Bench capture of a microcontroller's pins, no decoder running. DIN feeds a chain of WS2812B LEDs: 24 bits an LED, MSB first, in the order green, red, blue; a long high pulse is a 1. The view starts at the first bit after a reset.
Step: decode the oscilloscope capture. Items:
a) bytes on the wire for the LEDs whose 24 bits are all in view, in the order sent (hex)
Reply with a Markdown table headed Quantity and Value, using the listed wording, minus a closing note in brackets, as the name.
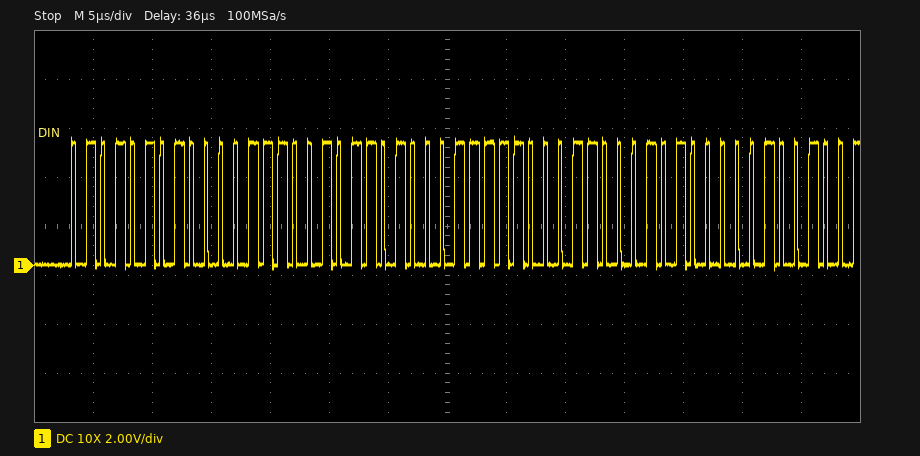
| Quantity | Value |
|---|---|
| bytes on the wire for the LEDs whose 24 bits are all in view, in the order sent | 55 0E 5A 3E 31 41 |
